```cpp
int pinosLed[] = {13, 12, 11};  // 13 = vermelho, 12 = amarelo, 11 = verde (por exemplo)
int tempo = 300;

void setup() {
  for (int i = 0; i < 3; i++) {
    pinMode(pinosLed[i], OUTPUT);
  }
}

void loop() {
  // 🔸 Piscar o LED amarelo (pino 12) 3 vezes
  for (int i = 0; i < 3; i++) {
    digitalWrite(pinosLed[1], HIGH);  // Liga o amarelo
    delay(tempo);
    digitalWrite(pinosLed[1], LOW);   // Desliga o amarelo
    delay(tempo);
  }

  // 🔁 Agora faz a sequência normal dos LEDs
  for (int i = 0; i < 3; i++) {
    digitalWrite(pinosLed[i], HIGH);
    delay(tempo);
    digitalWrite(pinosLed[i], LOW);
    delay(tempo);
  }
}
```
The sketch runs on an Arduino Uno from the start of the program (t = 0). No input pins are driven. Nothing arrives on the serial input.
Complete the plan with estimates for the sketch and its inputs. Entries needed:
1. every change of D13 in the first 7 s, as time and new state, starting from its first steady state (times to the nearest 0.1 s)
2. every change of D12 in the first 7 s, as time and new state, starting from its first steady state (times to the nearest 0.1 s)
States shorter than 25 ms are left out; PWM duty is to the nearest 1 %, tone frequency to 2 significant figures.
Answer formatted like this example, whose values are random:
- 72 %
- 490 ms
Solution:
- 0 s low; 1.8 s high; 2.1 s low; 5.4 s high; 5.7 s low
- 0 s high; 0.3 s low; 0.6 s high; 0.9 s low; 1.2 s high; 1.5 s low; 2.4 s high; 2.7 s low; 3.6 s high; 3.9 s low; 4.2 s high; 4.5 s low; 4.8 s high; 5.1 s low; 6 s high; 6.3 s low
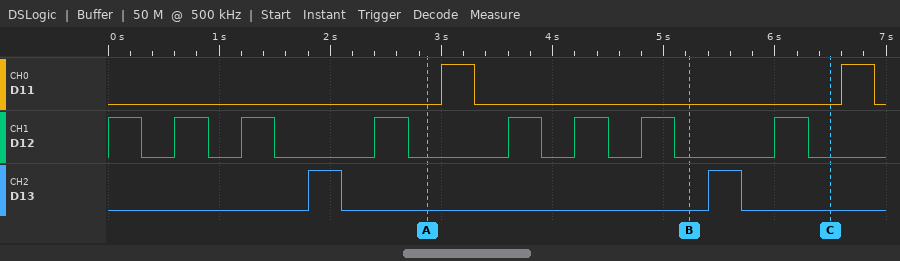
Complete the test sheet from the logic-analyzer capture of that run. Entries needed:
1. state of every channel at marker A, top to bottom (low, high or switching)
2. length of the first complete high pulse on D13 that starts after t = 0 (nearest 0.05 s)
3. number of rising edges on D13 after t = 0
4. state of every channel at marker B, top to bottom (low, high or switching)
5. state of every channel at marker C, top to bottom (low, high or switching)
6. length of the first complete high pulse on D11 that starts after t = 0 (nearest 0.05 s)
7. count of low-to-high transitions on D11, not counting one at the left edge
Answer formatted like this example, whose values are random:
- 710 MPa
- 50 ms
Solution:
- D11 low, D12 low, D13 low
- 0.30 s
- 2
- D11 low, D12 low, D13 low
- D11 low, D12 low, D13 low
- 0.30 s
- 2
